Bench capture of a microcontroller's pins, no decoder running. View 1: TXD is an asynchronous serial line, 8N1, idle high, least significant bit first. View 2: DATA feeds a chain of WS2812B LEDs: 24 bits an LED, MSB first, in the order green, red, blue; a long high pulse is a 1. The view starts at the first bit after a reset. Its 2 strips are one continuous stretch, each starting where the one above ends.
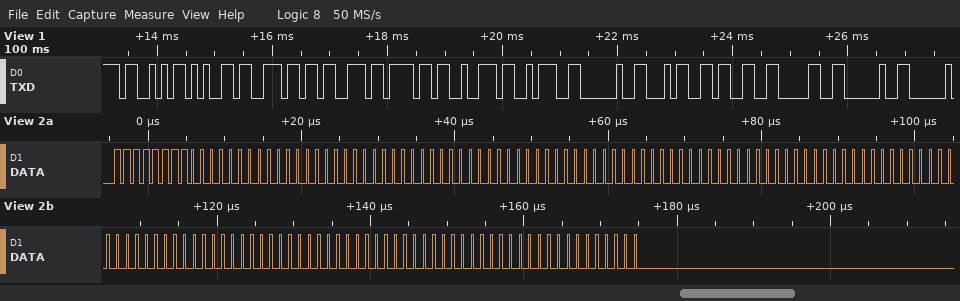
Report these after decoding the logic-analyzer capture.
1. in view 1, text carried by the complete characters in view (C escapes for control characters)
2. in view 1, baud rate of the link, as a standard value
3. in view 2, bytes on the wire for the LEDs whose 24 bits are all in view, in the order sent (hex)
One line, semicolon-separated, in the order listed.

"Sensor: 430 "; 9600 baud; FF 00 00 00 00 00 00 00 00 00 00 00 00 00 00 00 00 00
